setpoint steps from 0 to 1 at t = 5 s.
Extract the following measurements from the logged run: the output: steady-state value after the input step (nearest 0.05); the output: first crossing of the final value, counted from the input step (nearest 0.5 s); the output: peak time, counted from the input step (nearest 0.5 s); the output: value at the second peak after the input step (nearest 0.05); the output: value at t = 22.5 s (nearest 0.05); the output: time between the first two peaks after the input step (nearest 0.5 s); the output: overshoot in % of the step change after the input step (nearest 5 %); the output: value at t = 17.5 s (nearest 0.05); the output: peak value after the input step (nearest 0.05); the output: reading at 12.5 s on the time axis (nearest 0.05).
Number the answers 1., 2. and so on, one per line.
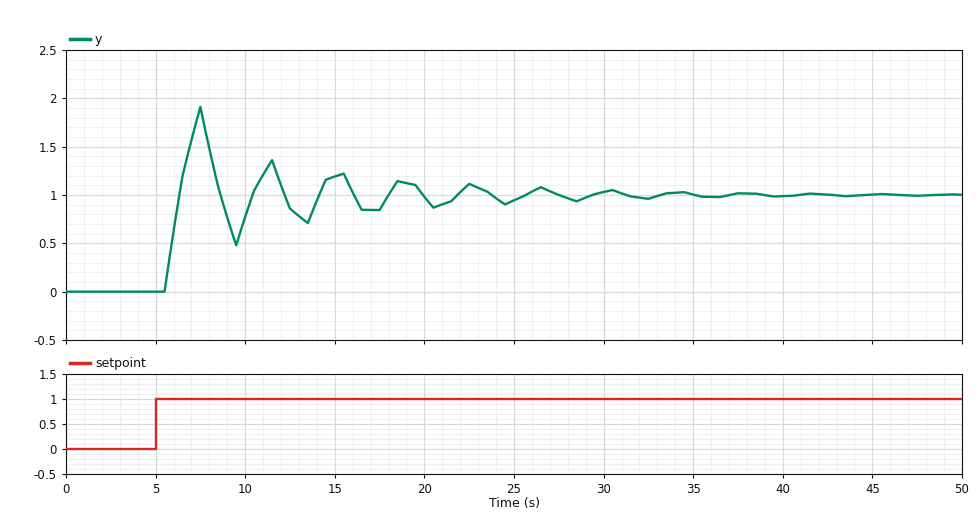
1. 1.00
2. 1.5 s
3. 2.5 s
4. 1.35
5. 1.10
6. 4.0 s
7. 90 %
8. 0.85
9. 1.90
10. 0.85
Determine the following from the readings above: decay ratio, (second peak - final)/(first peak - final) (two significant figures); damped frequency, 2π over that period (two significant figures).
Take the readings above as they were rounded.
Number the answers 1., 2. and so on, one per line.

1. 0.39
2. 1.6 rad/s
